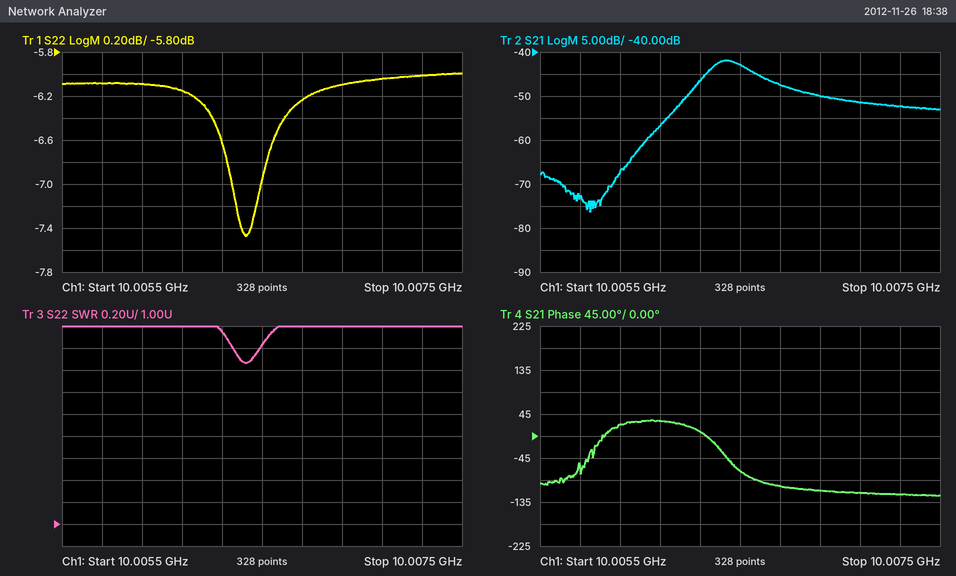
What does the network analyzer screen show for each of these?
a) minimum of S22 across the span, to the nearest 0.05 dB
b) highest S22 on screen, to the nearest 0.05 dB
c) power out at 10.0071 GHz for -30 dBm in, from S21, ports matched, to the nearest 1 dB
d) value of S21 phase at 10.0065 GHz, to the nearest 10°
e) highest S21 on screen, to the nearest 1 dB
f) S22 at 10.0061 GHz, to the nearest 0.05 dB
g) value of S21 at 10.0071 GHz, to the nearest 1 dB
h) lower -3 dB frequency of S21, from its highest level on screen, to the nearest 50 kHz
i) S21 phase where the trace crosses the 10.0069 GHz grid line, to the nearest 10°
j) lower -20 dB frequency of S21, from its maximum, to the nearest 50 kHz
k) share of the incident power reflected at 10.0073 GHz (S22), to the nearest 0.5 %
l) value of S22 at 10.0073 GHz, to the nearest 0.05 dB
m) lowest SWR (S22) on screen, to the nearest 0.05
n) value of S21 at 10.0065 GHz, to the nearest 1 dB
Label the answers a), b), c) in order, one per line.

a) -7.45 dB
b) -6.00 dB
c) -81 dBm
d) -70°
e) -42 dB
f) -6.15 dB
g) -51 dB
h) 10.00635 GHz
i) -110°
j) 10.00600 GHz
k) 25.0 %
l) -6.00 dB
m) 2.45
n) -43 dB
